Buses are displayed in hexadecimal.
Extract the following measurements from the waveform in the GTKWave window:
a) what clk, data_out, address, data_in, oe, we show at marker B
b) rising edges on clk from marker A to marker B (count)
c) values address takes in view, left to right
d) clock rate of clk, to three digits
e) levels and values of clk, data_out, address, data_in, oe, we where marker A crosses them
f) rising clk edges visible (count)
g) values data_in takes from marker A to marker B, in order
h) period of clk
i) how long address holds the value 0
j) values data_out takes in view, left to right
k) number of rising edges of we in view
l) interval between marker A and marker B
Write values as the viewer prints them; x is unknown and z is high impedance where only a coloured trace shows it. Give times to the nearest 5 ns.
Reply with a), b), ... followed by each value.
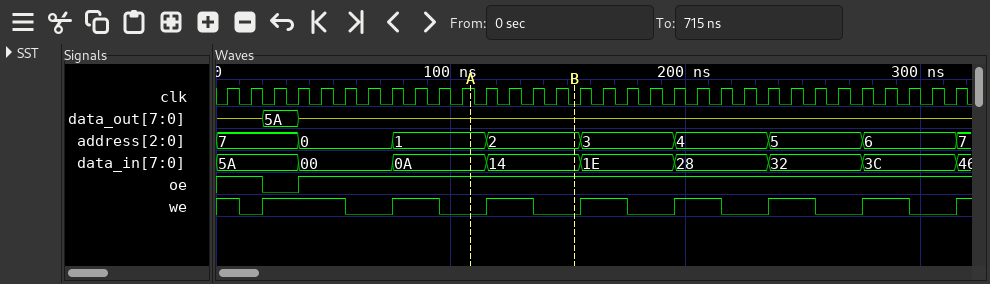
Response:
a) clk=0, data_out=z, address=2, data_in=14, oe=1, we=0
b) 4
c) 7, 0, 1, 2, 3, 4, 5, 6, 7
d) 100 MHz
e) clk=1, data_out=z, address=1, data_in=0A, oe=1, we=0
f) 32
g) 0A, 14
h) 10 ns
i) 40 ns
j) z, 5A, z
k) 8
l) 45 ns
